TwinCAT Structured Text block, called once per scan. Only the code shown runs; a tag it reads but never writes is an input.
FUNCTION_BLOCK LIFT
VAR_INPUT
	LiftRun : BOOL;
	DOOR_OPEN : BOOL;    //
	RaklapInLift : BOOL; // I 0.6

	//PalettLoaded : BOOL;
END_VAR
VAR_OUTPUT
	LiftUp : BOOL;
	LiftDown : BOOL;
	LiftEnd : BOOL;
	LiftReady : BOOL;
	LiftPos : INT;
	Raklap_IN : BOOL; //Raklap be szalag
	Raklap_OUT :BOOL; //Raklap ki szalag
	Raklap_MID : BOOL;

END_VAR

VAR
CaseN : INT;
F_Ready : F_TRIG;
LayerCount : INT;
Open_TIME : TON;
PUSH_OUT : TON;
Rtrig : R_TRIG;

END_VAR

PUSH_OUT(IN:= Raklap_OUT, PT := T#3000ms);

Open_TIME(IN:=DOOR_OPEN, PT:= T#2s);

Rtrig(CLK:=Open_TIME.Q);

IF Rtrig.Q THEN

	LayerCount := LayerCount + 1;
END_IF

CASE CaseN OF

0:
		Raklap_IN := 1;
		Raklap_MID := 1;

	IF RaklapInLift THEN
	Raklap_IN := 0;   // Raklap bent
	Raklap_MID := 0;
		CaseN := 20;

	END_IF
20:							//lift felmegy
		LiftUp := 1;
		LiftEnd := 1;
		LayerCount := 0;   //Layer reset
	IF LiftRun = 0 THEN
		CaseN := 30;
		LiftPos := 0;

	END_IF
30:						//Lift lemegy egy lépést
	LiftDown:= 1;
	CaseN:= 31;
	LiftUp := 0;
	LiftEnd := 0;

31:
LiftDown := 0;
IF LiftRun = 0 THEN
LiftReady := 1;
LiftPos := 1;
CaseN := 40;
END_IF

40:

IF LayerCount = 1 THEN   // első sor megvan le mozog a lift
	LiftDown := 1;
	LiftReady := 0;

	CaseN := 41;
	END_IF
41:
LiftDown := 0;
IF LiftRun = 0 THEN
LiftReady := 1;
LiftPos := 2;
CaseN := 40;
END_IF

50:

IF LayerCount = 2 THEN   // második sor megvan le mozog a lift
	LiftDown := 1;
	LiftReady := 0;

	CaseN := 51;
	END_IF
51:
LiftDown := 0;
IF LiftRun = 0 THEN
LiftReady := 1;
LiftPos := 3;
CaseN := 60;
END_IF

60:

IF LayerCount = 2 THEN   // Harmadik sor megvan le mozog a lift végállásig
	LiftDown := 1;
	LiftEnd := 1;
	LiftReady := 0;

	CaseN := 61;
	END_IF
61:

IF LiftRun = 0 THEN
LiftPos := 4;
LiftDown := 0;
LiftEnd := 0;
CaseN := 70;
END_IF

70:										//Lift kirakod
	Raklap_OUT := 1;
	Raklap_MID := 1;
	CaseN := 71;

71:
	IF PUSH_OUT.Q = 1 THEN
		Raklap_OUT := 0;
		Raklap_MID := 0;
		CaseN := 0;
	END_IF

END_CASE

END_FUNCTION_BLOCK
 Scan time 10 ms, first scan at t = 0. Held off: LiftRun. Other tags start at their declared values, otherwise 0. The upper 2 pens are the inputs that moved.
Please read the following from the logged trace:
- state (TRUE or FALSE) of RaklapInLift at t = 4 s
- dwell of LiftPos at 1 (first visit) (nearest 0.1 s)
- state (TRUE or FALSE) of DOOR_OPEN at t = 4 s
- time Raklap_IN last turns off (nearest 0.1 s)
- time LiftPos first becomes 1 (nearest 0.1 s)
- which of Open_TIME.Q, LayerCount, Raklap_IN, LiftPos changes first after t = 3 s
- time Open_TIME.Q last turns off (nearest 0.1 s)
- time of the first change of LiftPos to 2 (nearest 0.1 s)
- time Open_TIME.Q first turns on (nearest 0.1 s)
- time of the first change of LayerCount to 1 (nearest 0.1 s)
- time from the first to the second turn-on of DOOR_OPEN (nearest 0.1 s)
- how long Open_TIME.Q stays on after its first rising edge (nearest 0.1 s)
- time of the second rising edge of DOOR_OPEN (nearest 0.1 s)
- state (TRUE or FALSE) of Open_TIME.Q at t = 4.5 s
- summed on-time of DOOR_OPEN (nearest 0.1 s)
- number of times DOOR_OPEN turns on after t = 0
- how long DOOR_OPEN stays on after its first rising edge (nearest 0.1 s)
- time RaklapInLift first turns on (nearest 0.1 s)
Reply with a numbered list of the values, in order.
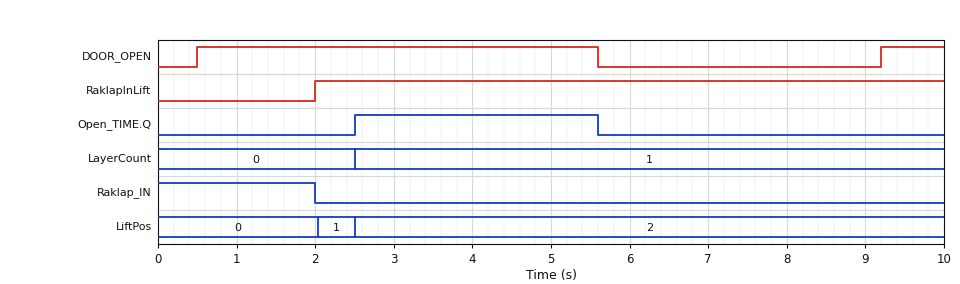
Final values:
1. TRUE
2. 0.5 s
3. TRUE
4. 2.0 s
5. 2.0 s
6. Open_TIME.Q
7. 5.6 s
8. 2.5 s
9. 2.5 s
10. 2.5 s
11. 8.7 s
12. 3.1 s
13. 9.2 s
14. TRUE
15. 5.9 s
16. 2
17. 5.1 s
18. 2.0 s
